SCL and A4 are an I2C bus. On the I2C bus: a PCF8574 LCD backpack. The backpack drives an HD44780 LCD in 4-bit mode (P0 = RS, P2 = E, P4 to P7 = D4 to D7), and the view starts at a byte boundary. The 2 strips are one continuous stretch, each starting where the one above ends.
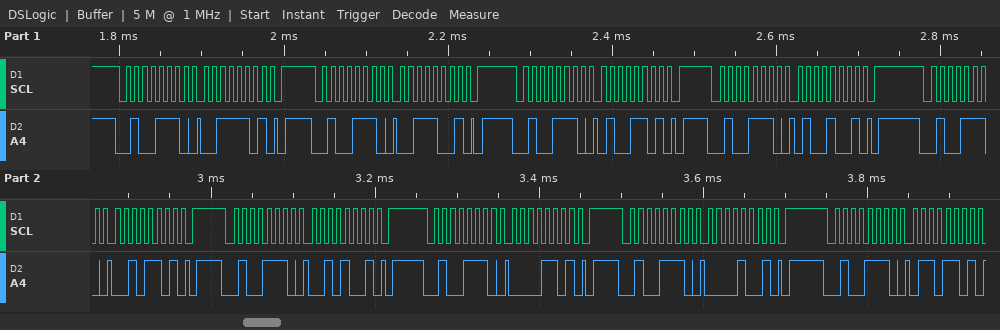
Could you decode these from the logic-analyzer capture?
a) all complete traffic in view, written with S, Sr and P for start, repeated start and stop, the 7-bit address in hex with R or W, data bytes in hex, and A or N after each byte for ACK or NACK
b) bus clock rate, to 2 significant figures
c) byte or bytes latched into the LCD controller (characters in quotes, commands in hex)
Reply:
S 27W A 3D A P S 27W A 39 A P S 27W A 4D A P S 27W A 49 A P S 27W A 2D A P S 27W A 29 A P S 27W A 0D A P S 27W A 09 A P S 27W A 6D A
100 kHz
'4' ' '
